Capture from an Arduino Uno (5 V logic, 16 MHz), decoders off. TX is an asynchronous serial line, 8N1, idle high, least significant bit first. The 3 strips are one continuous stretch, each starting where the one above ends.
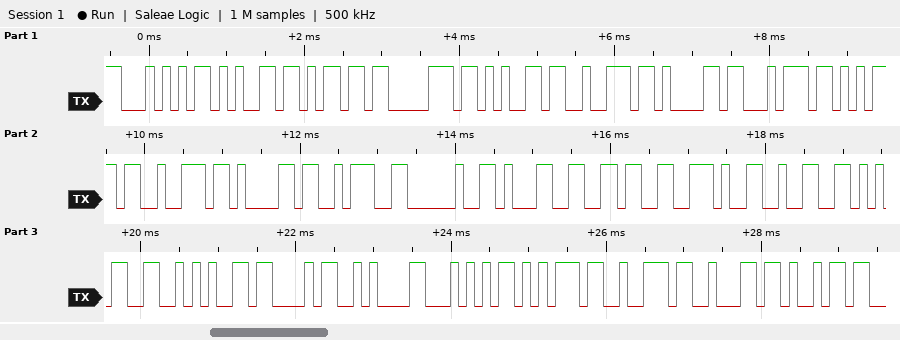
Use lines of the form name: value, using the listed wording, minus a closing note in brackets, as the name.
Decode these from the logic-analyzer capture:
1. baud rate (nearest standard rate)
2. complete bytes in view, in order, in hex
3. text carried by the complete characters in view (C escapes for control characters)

baud rate: 9600 baud
complete bytes in view, in order, in hex: 54 65 6D 70 65 72 61 74 75 72 61 3A 20 31 36 2E 32 35 2A 43 0A 54 75 72 62 69
text carried by the complete characters in view: "Temperatura: 16.25*C\nTurbi"
